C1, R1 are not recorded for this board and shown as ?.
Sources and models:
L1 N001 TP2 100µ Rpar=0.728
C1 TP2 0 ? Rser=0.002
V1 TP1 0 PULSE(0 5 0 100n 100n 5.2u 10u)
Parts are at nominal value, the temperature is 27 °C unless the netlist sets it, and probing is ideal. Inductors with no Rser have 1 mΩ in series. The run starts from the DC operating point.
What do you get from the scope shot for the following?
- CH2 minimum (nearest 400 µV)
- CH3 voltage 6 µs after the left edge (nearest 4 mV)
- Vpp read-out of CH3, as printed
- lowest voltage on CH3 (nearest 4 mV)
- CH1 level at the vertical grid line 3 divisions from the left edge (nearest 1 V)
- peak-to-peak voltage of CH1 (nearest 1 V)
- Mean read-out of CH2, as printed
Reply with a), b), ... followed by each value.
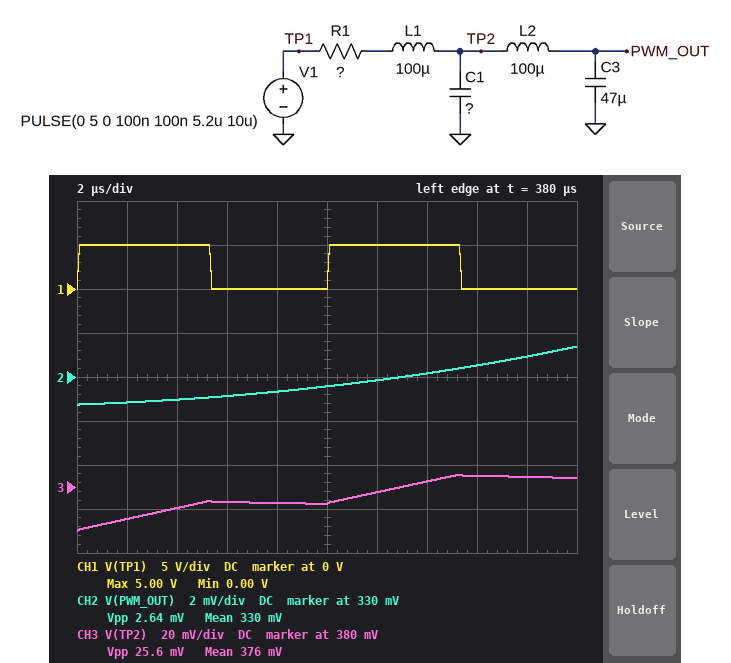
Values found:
a) 328.8 mV
b) 372 mV
c) 25.6 mV
d) 360 mV
e) 0 V
f) 5 V
g) 330 mV
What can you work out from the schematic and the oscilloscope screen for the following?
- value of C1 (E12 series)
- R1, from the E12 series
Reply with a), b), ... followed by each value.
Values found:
a) 100 µF
b) 18 Ω
